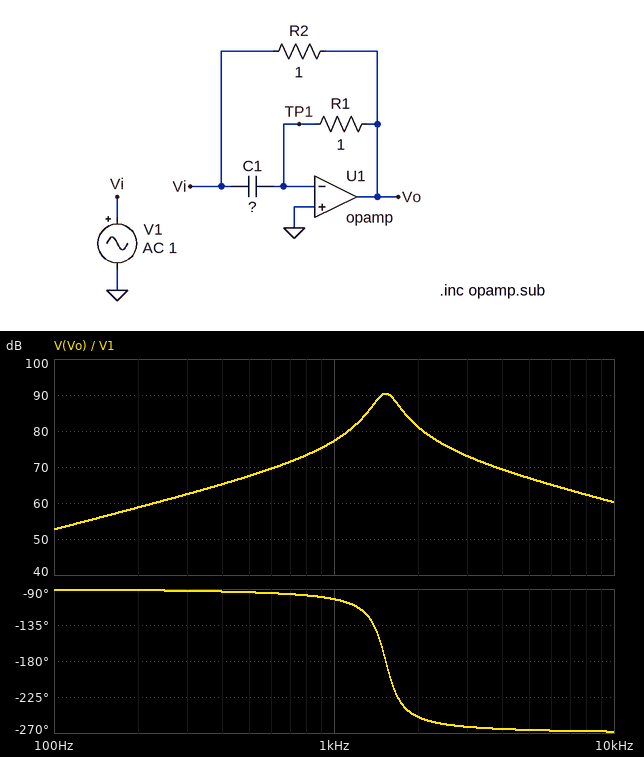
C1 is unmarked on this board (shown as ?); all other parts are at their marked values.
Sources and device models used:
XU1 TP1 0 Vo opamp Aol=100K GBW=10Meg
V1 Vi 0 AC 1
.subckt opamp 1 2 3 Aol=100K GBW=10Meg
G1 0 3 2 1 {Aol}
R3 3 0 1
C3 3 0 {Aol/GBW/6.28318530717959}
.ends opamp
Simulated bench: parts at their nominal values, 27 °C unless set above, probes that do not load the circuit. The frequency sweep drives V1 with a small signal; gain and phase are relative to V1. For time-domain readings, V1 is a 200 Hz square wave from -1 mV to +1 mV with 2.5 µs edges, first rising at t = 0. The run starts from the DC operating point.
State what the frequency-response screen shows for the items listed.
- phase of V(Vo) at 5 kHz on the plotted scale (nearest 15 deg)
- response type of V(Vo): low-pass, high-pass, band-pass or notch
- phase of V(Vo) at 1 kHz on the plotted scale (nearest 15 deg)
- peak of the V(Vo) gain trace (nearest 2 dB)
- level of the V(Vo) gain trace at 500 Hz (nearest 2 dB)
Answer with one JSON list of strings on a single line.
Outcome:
["-270 deg", "band-pass", "-105 deg", "90 dB", "68 dB"]
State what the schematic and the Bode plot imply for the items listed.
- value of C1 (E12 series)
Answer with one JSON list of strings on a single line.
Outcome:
["680 mF"]
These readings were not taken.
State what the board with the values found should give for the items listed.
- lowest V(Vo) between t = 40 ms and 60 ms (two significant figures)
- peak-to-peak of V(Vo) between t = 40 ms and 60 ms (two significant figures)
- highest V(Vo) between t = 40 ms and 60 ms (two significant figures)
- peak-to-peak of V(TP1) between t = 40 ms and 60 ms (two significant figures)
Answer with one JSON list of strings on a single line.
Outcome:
["-11 V", "22 V", "11 V", "3.9 mV"]
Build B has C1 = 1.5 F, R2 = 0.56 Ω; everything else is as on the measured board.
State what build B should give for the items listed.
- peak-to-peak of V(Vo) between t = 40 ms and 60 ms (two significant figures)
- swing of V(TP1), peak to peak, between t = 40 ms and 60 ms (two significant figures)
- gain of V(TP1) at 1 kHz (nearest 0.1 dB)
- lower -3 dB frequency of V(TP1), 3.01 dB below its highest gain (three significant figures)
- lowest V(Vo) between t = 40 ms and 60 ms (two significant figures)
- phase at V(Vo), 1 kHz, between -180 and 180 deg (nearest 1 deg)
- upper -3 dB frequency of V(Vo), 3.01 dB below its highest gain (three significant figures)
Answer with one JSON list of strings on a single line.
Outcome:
["32 V", "4.2 mV", "8.9 dB", "900 Hz", "-16 V", "-171 deg", "1.24 kHz"]
